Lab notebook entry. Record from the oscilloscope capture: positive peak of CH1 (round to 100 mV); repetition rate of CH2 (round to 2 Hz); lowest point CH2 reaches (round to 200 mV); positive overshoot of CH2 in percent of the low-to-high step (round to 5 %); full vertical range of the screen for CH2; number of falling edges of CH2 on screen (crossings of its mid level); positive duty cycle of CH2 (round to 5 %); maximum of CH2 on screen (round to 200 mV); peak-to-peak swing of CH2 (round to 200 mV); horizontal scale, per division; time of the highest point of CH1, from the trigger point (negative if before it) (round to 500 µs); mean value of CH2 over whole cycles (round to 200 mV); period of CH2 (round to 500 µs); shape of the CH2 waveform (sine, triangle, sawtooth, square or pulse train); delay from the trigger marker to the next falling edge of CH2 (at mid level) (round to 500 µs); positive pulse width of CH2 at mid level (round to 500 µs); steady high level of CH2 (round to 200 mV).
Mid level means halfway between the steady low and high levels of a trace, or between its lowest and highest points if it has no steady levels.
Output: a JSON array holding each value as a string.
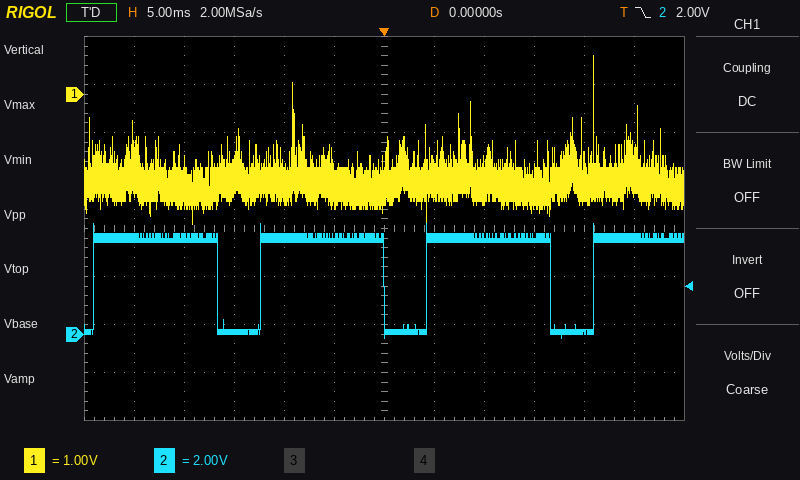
["800 mV", "60 Hz", "-200 mV", "15 %", "16 V", "3", "75 %", "4.6 V", "4.8 V", "5 ms", "+21.0 ms", "3.0 V", "16.5 ms", "pulse train", "16.5 ms", "12.5 ms", "4.0 V"]
